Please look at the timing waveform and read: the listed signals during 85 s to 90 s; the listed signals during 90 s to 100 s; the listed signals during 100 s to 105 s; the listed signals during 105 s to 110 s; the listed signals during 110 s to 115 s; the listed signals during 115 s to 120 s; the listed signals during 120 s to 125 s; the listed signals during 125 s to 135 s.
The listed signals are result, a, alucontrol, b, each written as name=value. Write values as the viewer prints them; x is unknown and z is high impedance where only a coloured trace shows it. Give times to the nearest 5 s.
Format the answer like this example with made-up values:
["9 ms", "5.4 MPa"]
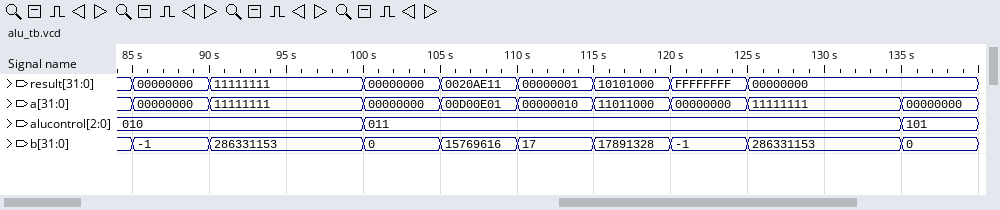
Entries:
["result=00000000, a=00000000, alucontrol=010, b=-1", "result=11111111, a=11111111, alucontrol=010, b=286331153", "result=00000000, a=00000000, alucontrol=011, b=0", "result=0020AE11, a=00D00E01, alucontrol=011, b=15769616", "result=00000001, a=00000010, alucontrol=011, b=17", "result=10101000, a=11011000, alucontrol=011, b=17891328", "result=FFFFFFFF, a=00000000, alucontrol=011, b=-1", "result=00000000, a=11111111, alucontrol=011, b=286331153"]
